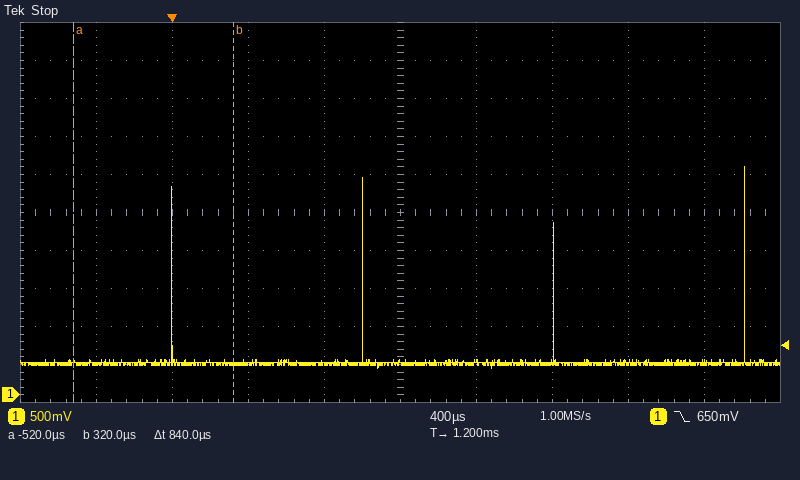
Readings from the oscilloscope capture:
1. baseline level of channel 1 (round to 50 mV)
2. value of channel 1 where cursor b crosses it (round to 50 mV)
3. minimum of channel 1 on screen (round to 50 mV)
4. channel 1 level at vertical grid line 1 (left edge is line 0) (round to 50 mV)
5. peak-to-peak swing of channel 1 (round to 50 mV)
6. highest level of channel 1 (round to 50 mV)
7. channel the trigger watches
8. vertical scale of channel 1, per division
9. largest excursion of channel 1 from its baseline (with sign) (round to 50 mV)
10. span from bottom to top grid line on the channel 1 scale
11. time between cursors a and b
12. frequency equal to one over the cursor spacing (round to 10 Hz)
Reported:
400 mV
400 mV
350 mV
400 mV
2.65 V
3.00 V
channel 1
500 mV
+2.60 V
5 V
840 µs
1.19 kHz
